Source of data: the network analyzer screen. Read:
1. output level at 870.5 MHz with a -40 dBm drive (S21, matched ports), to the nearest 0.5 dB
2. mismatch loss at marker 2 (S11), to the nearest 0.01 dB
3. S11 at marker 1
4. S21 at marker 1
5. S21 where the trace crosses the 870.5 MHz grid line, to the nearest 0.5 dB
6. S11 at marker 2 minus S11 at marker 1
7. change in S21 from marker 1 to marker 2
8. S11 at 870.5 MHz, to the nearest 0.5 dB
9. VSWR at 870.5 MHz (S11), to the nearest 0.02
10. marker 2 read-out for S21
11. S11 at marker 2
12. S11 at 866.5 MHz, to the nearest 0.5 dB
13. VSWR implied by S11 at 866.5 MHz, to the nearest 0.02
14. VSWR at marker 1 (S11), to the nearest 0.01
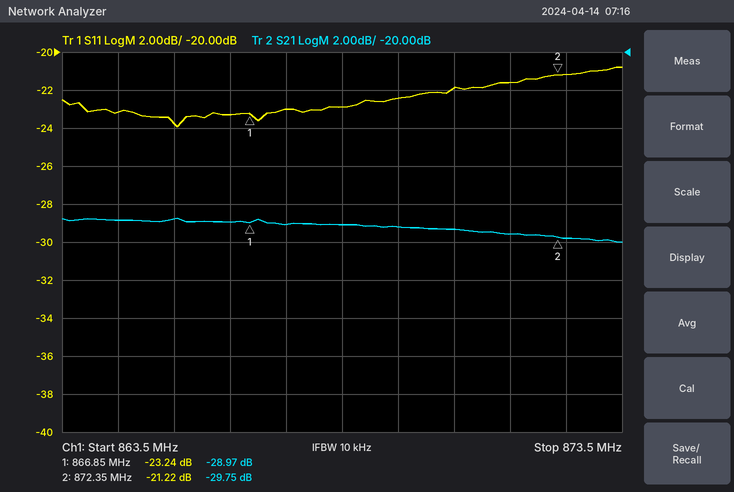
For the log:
-69.5 dBm
0.03 dB
-23.24 dB
-28.97 dB
-29.5 dB
2.02 dB
-0.78 dB
-22.0 dB
1.18
-29.75 dB
-21.22 dB
-23.5 dB
1.14
1.15
